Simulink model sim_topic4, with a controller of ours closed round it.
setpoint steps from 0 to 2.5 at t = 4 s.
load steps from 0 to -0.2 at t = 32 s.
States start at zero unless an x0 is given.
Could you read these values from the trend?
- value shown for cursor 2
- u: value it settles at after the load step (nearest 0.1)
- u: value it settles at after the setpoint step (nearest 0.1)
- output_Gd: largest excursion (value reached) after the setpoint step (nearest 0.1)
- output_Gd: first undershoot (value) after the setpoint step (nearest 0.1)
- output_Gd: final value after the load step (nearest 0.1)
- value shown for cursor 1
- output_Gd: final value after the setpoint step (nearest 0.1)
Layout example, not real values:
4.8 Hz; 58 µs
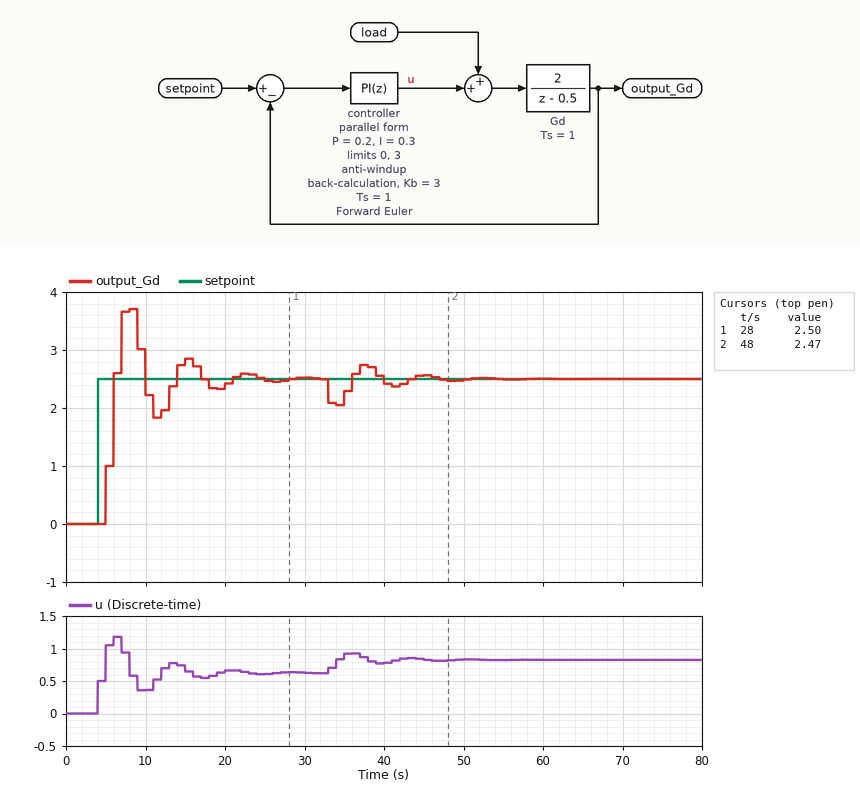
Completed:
2.47; 0.8; 0.6; 3.7; 1.8; 2.5; 2.50; 2.5
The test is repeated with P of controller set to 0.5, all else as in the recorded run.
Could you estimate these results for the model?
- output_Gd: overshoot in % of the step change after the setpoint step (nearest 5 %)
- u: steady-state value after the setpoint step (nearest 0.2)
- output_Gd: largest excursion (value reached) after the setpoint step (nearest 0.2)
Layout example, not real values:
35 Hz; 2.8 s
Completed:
10 %; 0.6; 2.8
